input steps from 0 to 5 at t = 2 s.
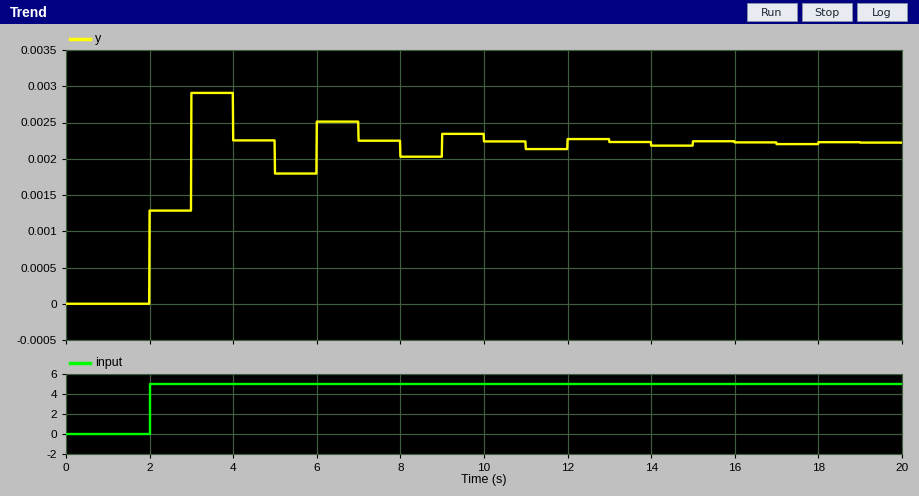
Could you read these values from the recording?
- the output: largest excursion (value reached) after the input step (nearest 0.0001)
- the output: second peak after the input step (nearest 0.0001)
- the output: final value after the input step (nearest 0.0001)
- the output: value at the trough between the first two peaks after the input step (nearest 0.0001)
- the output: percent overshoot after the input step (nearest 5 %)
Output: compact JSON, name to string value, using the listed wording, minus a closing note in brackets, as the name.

{"the output: largest excursion (value reached) after the input step": "0.0029", "the output: second peak after the input step": "0.0025", "the output: final value after the input step": "0.0022", "the output: value at the trough between the first two peaks after the input step": "0.0018", "the output: percent overshoot after the input step": "30 %"}
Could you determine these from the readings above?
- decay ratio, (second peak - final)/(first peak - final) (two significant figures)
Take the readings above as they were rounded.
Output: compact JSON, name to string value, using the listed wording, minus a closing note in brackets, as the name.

{"decay ratio, (second peak - final)/(first peak - final)": "0.43"}
